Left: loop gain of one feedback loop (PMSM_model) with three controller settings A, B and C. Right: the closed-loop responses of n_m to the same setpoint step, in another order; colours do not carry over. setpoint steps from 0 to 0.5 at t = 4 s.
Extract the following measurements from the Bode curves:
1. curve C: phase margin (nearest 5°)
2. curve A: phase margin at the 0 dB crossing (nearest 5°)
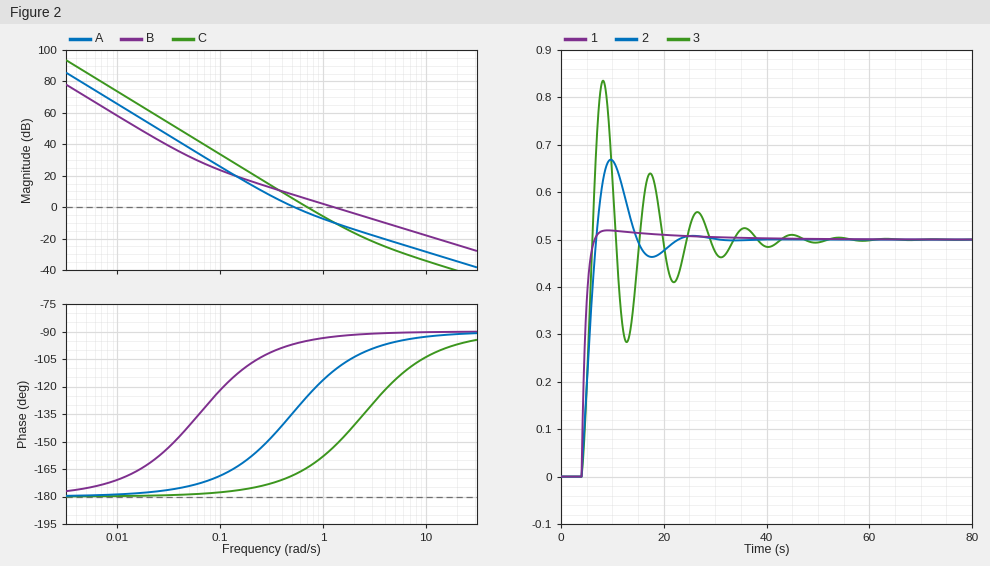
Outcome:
15°
45°
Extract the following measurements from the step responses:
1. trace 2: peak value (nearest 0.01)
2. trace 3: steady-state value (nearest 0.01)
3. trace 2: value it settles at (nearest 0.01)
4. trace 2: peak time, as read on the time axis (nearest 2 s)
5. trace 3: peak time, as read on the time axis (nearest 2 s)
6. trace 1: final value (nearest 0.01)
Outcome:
0.67
0.50
0.50
10 s
8 s
0.50
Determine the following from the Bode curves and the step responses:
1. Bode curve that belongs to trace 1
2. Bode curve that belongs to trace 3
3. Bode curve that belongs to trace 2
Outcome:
B
C
A
